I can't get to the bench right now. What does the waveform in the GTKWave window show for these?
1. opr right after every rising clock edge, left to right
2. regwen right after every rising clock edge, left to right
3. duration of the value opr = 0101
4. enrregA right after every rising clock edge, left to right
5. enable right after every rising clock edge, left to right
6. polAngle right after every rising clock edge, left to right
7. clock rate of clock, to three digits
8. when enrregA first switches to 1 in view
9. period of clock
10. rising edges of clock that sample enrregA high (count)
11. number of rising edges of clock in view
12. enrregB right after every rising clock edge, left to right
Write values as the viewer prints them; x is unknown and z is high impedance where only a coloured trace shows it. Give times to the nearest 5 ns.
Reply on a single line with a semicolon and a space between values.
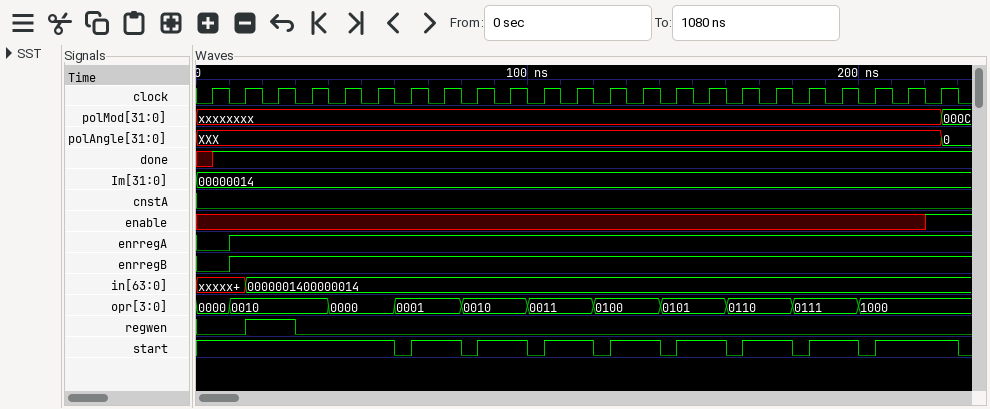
0000, 0010, 0010, 0010, 0000, 0000, 0001, 0001, 0010, 0010, 0011, 0011, 0100, 0100, 0101, 0101, 0110, 0110, 0111, 0111, 1000, 1000, 1000; 0 1 1 0 0 0 0 0 0 0 0 0 0 0 0 0 0 0 0 0 0 0 0; 20 ns; 0 1 1 1 1 1 1 1 1 1 1 1 1 1 1 1 1 1 1 1 1 1 1; x x x x x x x x x x x x x x x x x x x x x x 1; XXX, XXX, XXX, XXX, XXX, XXX, XXX, XXX, XXX, XXX, XXX, XXX, XXX, XXX, XXX, XXX, XXX, XXX, XXX, XXX, XXX, XXX, 0; 100 MHz; 10 ns; 10 ns; 22; 23; 0 1 1 1 1 1 1 1 1 1 1 1 1 1 1 1 1 1 1 1 1 1 1
